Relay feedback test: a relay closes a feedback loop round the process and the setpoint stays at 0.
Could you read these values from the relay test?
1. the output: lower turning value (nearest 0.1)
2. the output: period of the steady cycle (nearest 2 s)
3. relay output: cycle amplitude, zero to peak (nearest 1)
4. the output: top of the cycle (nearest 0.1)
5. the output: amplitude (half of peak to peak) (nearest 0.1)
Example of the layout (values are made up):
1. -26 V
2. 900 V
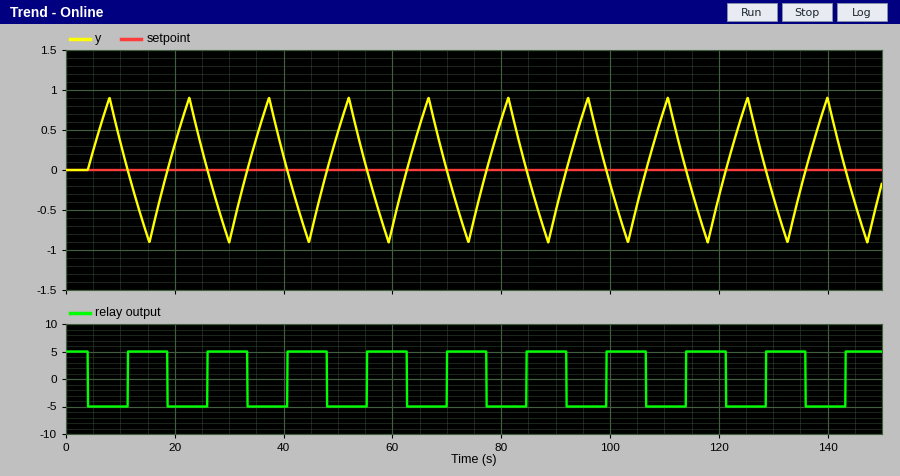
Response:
1. -0.9
2. 14 s
3. 5
4. 0.9
5. 0.9
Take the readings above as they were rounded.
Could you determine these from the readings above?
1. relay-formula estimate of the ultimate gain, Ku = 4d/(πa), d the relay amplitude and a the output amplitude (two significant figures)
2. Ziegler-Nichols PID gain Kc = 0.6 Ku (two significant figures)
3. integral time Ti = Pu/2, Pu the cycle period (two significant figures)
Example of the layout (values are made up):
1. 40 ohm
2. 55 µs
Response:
1. 7.1
2. 4.3
3. 7.0 s
